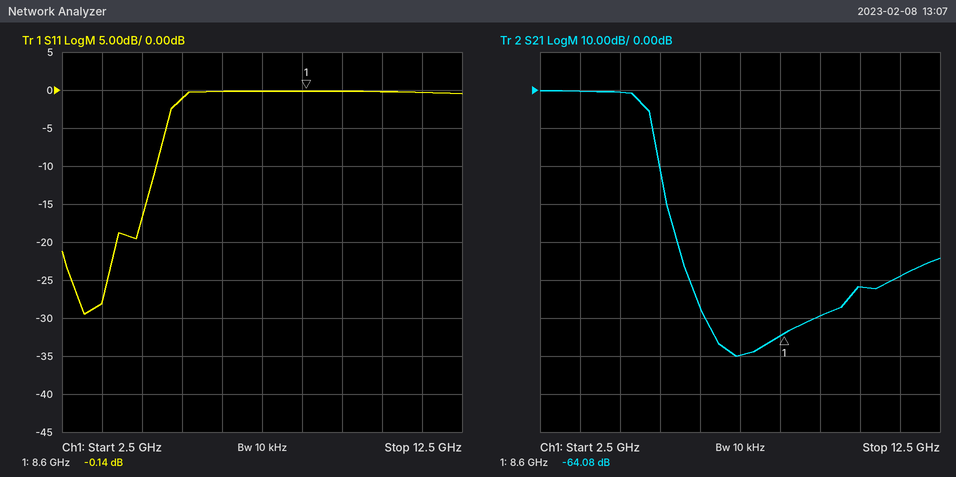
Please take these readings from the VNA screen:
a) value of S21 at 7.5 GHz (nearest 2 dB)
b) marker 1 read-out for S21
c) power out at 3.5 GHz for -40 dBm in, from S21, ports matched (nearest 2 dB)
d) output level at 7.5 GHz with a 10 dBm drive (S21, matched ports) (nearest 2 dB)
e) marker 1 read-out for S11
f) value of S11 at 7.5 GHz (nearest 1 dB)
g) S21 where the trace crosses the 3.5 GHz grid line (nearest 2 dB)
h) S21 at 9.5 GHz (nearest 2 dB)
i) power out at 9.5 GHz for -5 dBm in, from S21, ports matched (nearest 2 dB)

-70 dB
-64.08 dB
-40 dBm
-60 dBm
-0.14 dB
0 dB
0 dB
-60 dB
-64 dBm
